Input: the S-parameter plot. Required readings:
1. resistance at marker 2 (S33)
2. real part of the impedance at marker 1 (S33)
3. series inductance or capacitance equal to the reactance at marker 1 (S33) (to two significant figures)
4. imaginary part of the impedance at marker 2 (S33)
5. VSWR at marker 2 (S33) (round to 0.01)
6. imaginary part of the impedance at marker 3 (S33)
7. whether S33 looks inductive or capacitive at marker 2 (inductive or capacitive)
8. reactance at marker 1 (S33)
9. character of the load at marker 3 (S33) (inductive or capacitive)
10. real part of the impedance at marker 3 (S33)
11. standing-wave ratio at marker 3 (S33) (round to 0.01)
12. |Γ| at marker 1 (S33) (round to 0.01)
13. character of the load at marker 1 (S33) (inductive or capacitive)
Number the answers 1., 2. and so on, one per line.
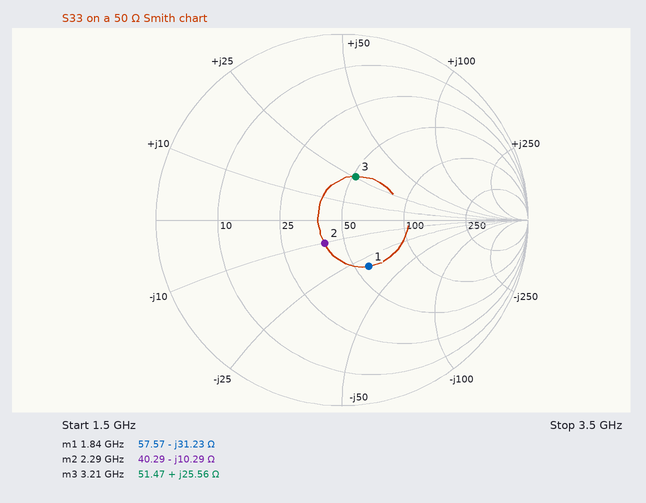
1. 40.29 Ω
2. 57.57 Ω
3. 2.8 pF
4. -10.29 Ω
5. 1.37
6. +25.56 Ω
7. capacitive
8. -31.23 Ω
9. inductive
10. 51.47 Ω
11. 1.65
12. 0.29
13. capacitive
